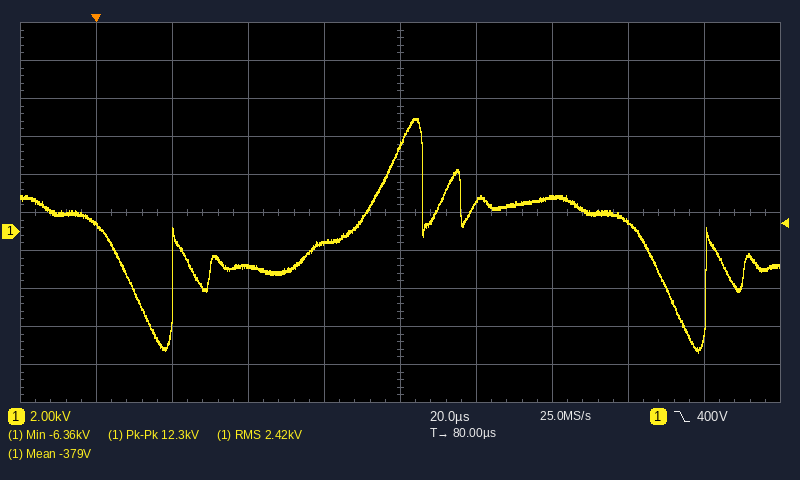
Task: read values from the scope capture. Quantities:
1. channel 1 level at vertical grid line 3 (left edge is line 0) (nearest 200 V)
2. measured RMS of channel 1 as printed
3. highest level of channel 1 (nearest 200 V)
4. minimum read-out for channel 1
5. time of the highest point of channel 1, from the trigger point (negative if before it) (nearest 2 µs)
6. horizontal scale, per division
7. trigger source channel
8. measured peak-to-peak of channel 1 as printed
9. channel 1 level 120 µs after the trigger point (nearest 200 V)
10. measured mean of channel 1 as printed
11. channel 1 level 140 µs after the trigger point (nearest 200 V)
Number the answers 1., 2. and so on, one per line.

1. -1.8 kV
2. 2.42 kV
3. 6.0 kV
4. -6.36 kV
5. +84 µs
6. 20 µs
7. channel 1
8. 12.3 kV
9. 1.8 kV
10. -379 V
11. 400 V
